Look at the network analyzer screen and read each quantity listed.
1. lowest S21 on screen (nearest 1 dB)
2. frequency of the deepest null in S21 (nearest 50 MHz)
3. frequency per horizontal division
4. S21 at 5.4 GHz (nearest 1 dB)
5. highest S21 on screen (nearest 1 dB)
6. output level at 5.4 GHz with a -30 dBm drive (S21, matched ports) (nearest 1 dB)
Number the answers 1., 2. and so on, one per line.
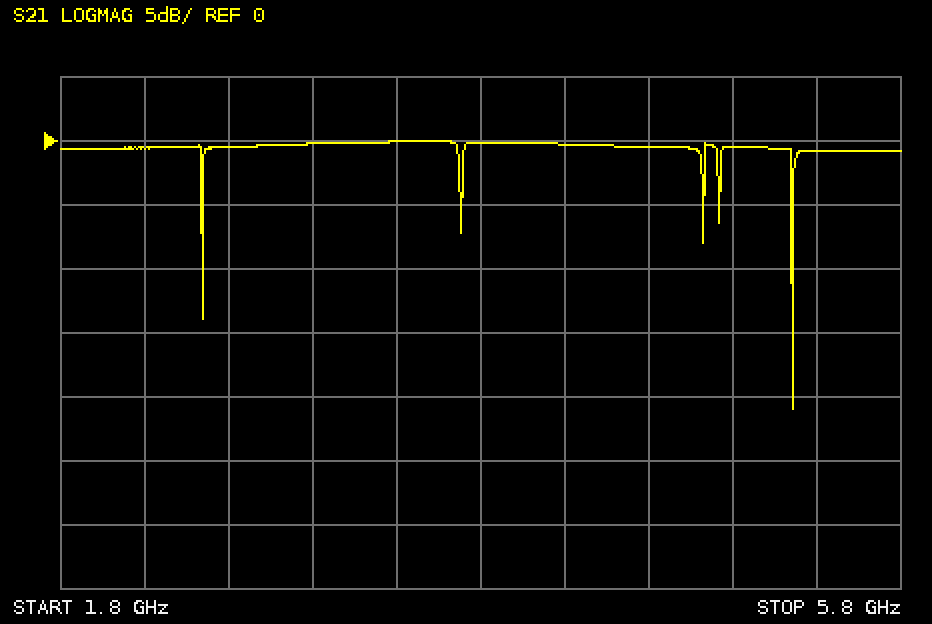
1. -21 dB
2. 5.30 GHz
3. 400 MHz
4. -1 dB
5. 0 dB
6. -31 dBm
